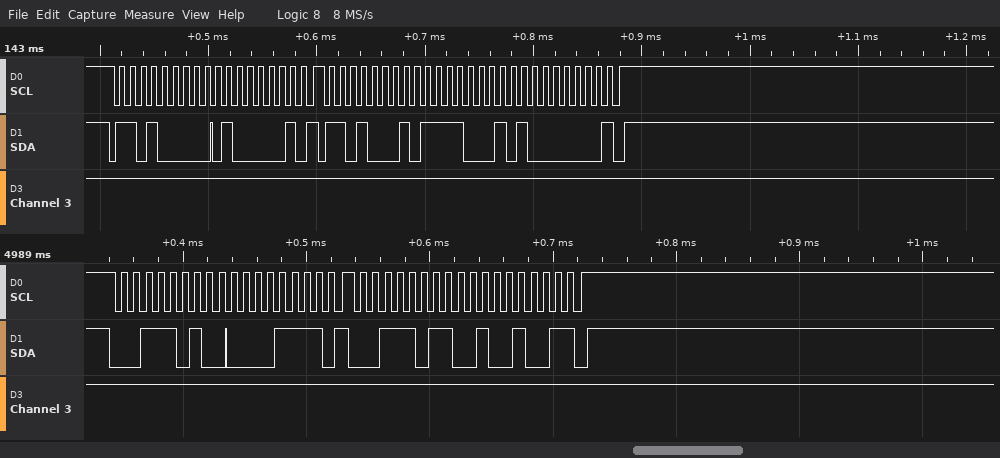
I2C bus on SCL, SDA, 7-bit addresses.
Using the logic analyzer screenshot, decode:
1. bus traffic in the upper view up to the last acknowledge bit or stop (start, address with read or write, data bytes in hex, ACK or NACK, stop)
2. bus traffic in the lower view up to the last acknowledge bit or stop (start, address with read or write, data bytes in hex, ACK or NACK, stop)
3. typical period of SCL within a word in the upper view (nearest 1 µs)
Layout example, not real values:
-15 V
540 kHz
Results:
start, address 68 write ACK, 41 ACK, repeated start, address 68 read ACK, F1 ACK, 80 NACK, stop
start, address 1D write ACK, 0F ACK, repeated start, address 1D read ACK, 49 NACK, stop
10 µs
